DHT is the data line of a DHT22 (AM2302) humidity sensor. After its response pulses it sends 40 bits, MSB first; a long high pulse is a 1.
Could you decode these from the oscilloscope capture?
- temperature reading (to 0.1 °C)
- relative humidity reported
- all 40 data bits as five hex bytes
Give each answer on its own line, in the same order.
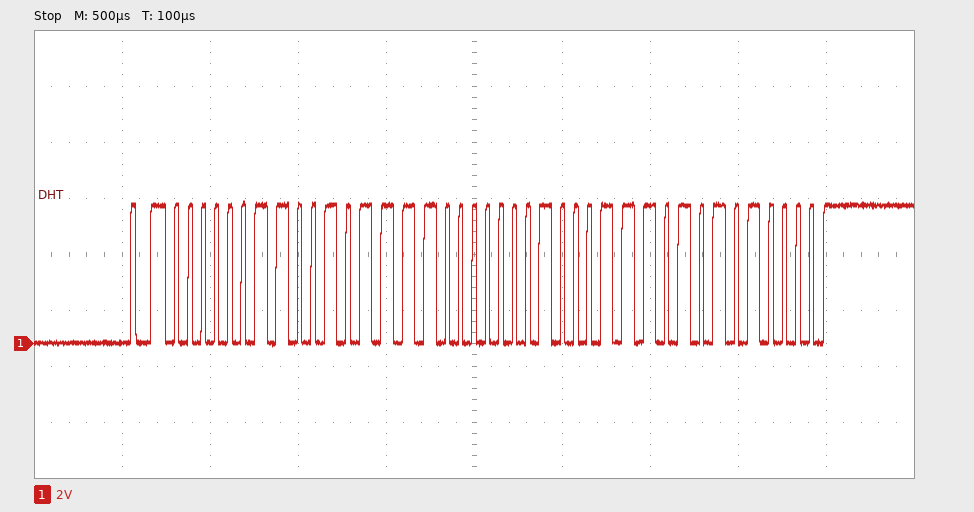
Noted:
28.5 °C
81.5 %
03 2F 01 1D 50
